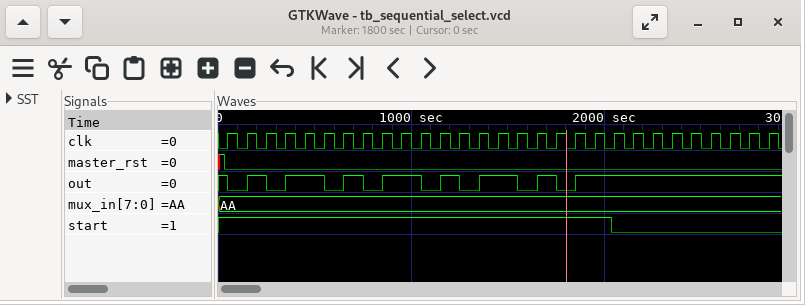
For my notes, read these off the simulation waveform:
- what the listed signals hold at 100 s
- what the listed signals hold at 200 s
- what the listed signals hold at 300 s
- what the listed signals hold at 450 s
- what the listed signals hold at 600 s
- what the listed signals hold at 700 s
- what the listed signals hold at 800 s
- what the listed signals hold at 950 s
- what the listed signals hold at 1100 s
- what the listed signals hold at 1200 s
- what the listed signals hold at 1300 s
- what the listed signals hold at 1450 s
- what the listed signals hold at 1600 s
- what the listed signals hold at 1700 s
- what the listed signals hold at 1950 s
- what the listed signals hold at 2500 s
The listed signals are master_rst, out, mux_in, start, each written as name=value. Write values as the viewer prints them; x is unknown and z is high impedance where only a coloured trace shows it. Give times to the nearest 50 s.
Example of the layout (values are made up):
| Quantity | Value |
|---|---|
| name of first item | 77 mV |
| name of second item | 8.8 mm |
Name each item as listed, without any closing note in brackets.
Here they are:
| Quantity | Value |
|---|---|
| what the listed signals hold at 100 s | master_rst=0, out=0, mux_in=AA, start=1 |
| what the listed signals hold at 200 s | master_rst=0, out=1, mux_in=AA, start=1 |
| what the listed signals hold at 300 s | master_rst=0, out=0, mux_in=AA, start=1 |
| what the listed signals hold at 450 s | master_rst=0, out=1, mux_in=AA, start=1 |
| what the listed signals hold at 600 s | master_rst=0, out=0, mux_in=AA, start=1 |
| what the listed signals hold at 700 s | master_rst=0, out=1, mux_in=AA, start=1 |
| what the listed signals hold at 800 s | master_rst=0, out=0, mux_in=AA, start=1 |
| what the listed signals hold at 950 s | master_rst=0, out=1, mux_in=AA, start=1 |
| what the listed signals hold at 1100 s | master_rst=0, out=0, mux_in=AA, start=1 |
| what the listed signals hold at 1200 s | master_rst=0, out=1, mux_in=AA, start=1 |
| what the listed signals hold at 1300 s | master_rst=0, out=0, mux_in=AA, start=1 |
| what the listed signals hold at 1450 s | master_rst=0, out=1, mux_in=AA, start=1 |
| what the listed signals hold at 1600 s | master_rst=0, out=0, mux_in=AA, start=1 |
| what the listed signals hold at 1700 s | master_rst=0, out=1, mux_in=AA, start=1 |
| what the listed signals hold at 1950 s | master_rst=0, out=1, mux_in=AA, start=1 |
| what the listed signals hold at 2500 s | master_rst=0, out=1, mux_in=AA, start=0 |
